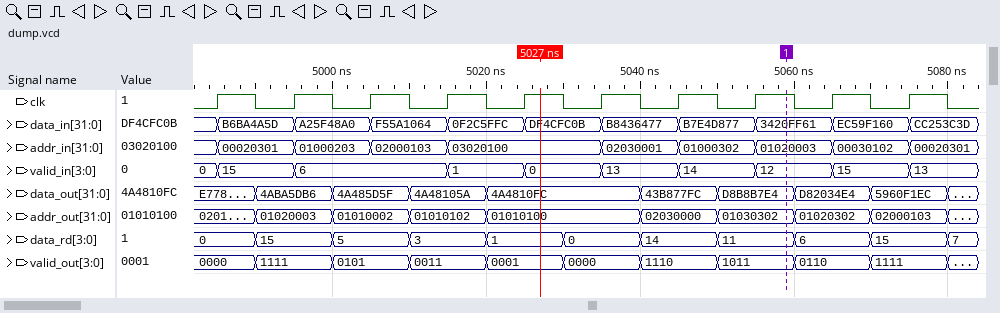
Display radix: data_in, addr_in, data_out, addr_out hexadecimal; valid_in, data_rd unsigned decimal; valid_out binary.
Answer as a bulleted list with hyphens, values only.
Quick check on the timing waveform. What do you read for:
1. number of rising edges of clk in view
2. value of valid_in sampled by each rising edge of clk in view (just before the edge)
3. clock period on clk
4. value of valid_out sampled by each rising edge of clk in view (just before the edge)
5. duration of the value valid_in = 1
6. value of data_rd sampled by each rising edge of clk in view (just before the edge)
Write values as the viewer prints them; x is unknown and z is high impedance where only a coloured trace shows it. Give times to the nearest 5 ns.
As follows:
- 10
- 0, 15, 6, 6, 1, 0, 13, 14, 12, 15
- 10 ns
- 0000, 1111, 0101, 0011, 0001, 0000, 1110, 1011, 0110, 1111
- 10 ns
- 0, 15, 5, 3, 1, 0, 14, 11, 6, 15
